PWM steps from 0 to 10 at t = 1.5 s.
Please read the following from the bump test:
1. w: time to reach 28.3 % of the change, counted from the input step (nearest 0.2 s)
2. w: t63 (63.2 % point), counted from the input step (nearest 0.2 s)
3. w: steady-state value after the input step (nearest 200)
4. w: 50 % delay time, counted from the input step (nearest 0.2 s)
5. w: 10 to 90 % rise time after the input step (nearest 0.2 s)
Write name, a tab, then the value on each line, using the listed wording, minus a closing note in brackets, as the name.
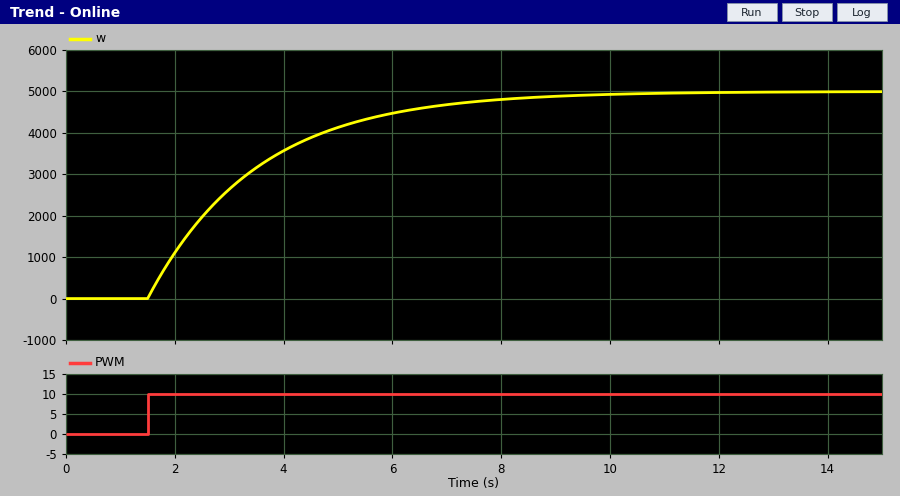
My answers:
w: time to reach 28.3 % of the change, counted from the input step	0.6 s
w: t63 (63.2 % point), counted from the input step	2.0 s
w: steady-state value after the input step	5000
w: 50 % delay time, counted from the input step	1.4 s
w: 10 to 90 % rise time after the input step	4.4 s
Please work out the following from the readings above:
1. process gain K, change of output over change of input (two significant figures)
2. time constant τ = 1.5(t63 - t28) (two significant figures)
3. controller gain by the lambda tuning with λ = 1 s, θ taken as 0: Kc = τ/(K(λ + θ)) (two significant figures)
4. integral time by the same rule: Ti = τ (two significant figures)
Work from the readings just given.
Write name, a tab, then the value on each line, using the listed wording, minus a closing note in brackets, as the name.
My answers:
process gain K, change of output over change of input	500
time constant τ = 1.5(t63 - t28)	2.1 s
controller gain by the lambda tuning with λ = 1 s, θ taken as 0: Kc = τ/(K(λ + θ))	0.0042
integral time by the same rule: Ti = τ	2.1 s
